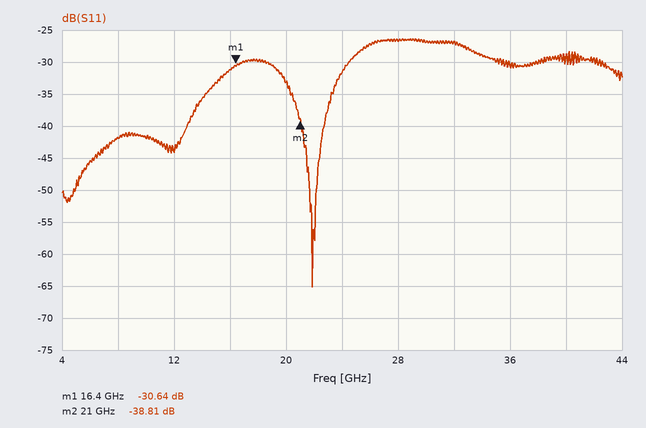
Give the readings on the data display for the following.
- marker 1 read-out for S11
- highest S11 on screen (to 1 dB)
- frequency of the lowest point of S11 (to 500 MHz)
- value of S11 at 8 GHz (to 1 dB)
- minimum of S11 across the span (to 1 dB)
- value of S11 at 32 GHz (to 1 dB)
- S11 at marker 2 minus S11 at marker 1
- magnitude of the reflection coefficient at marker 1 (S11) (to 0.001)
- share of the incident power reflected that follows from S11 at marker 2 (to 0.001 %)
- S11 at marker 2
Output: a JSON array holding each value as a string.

["-30.64 dB", "-26 dB", "22.0 GHz", "-42 dB", "-65 dB", "-27 dB", "-8.17 dB", "0.029", "0.013 %", "-38.81 dB"]
